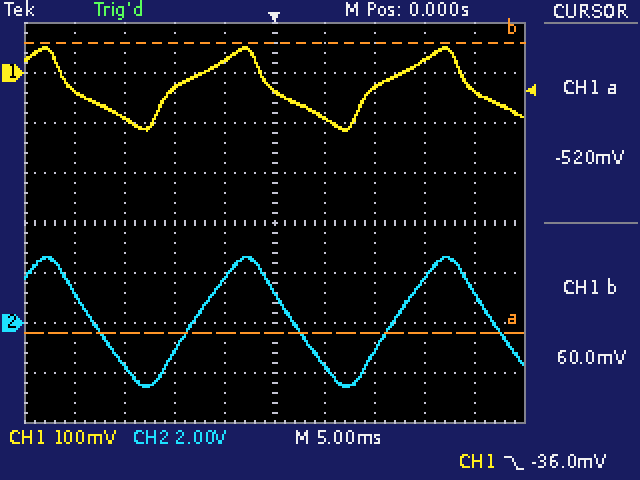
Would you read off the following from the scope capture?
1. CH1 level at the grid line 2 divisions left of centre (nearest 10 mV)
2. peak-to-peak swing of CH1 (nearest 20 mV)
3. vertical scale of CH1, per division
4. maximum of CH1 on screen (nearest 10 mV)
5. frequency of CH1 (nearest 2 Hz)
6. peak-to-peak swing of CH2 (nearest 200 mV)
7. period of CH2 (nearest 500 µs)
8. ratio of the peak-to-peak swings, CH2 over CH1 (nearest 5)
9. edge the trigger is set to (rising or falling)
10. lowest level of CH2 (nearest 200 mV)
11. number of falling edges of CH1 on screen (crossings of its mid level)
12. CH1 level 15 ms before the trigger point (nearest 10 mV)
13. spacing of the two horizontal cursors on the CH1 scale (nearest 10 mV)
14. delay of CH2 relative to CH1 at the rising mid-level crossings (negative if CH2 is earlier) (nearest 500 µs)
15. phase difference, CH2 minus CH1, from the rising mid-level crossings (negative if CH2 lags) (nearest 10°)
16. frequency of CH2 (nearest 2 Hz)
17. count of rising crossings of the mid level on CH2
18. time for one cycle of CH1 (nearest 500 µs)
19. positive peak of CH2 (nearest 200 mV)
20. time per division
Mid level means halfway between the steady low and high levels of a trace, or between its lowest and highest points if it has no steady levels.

-30 mV
160 mV
100 mV
50 mV
50 Hz
5.2 V
20.0 ms
30
falling
-2.6 V
3
-90 mV
580 mV
+2.0 ms
-40°
50 Hz
2
20.0 ms
2.6 V
5 ms
